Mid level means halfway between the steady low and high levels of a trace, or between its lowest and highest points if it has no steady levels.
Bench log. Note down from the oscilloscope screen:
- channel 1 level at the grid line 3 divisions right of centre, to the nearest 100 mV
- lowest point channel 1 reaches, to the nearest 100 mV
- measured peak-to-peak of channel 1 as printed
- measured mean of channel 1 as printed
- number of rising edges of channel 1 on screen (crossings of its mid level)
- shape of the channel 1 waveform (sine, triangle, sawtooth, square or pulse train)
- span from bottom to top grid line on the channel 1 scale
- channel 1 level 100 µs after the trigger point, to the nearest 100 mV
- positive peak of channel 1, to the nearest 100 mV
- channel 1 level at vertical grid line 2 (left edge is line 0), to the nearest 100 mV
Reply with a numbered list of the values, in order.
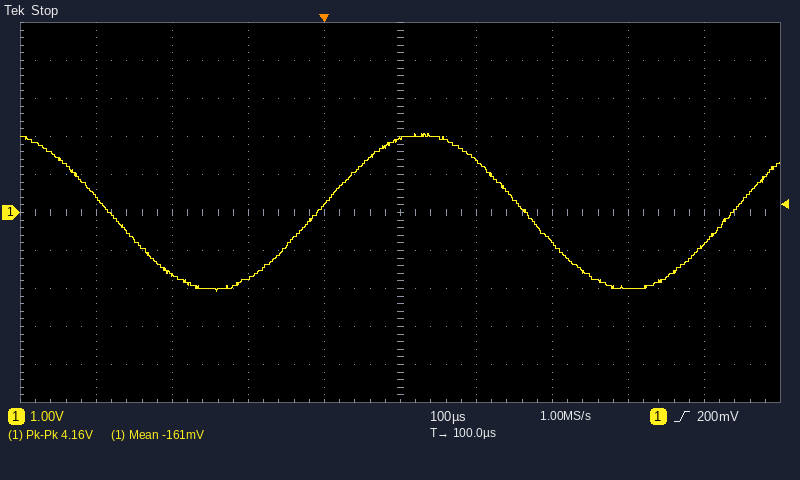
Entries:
1. -2.0 V
2. -2.1 V
3. 4.16 V
4. -161 mV
5. 2
6. sine
7. 10 V
8. 1.9 V
9. 2.1 V
10. -1.6 V
